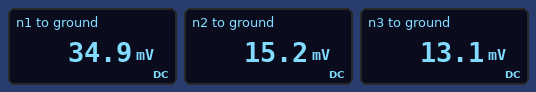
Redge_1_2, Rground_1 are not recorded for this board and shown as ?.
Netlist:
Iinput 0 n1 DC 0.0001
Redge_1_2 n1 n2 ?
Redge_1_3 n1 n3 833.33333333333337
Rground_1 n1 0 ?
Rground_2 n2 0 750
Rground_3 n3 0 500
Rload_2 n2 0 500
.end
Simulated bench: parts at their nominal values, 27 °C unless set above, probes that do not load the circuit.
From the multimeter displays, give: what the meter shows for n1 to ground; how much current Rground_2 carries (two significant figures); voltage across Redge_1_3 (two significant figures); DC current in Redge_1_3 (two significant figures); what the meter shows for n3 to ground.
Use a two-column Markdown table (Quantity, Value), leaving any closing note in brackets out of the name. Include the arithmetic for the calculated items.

| Quantity | Value |
|---|---|
| what the meter shows for n1 to ground | 34.9 mV |
| how much current Rground_2 carries | (15.2 mV) / 750 Ω = 20 µA |
| voltage across Redge_1_3 | 34.9 mV - 13.1 mV = 22 mV |
| DC current in Redge_1_3 | (34.9 mV - 13.1 mV) / 833.3 Ω = 26 µA |
| what the meter shows for n3 to ground | 13.1 mV |
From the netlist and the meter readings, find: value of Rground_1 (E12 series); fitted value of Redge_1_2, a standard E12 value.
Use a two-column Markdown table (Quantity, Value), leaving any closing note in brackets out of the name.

| Quantity | Value |
|---|---|
| value of Rground_1 | 1.5 kΩ |
| fitted value of Redge_1_2, a standard E12 value | 390 Ω |
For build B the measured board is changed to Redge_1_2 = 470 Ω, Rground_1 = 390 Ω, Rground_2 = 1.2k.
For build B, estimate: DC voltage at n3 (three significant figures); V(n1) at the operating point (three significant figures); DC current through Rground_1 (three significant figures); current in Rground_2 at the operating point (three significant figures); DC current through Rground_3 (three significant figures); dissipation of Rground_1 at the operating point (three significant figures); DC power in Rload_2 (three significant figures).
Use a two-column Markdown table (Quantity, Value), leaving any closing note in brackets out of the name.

| Quantity | Value |
|---|---|
| DC voltage at n3 | 8.28 mV |
| V(n1) at the operating point | 22.1 mV |
| DC current through Rground_1 | 56.6 µA |
| current in Rground_2 at the operating point | 7.89 µA |
| DC current through Rground_3 | 16.6 µA |
| dissipation of Rground_1 at the operating point | 1.25 µW |
| DC power in Rload_2 | 179 nW |
